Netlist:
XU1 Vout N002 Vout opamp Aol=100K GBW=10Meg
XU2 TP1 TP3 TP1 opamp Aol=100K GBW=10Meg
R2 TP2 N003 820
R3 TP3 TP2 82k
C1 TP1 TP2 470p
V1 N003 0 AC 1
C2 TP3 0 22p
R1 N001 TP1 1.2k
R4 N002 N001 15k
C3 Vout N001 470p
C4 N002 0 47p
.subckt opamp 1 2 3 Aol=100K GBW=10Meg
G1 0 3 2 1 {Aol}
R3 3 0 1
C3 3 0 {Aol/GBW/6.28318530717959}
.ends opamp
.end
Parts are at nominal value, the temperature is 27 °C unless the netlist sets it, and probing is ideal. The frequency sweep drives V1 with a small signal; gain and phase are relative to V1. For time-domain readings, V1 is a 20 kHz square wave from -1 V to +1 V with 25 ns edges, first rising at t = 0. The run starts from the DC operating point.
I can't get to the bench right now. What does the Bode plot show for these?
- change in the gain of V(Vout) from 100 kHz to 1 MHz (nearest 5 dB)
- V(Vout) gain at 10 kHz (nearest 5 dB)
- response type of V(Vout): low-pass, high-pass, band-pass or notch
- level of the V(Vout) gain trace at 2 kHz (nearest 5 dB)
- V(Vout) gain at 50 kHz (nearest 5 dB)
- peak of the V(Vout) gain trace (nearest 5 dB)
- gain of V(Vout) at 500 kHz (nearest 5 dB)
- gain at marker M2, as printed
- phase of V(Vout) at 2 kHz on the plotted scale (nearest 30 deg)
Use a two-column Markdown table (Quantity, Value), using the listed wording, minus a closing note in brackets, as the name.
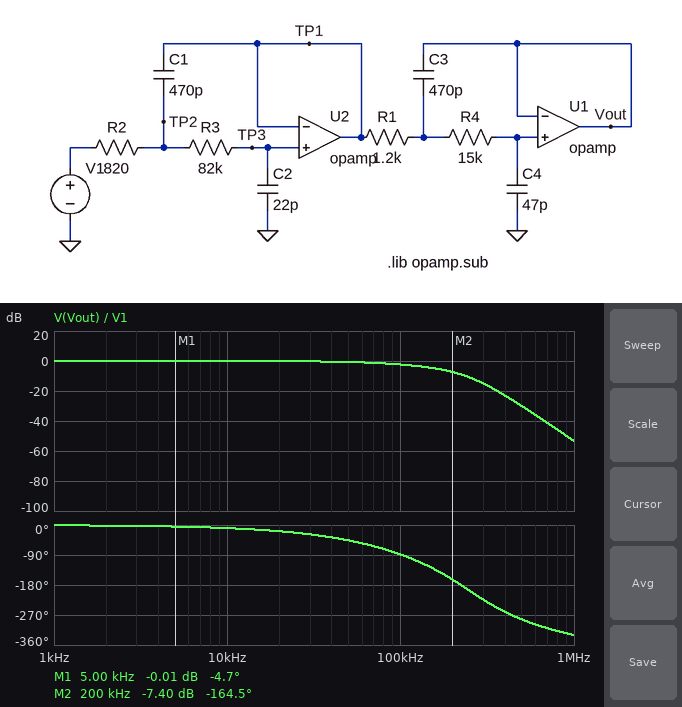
| Quantity | Value |
|---|---|
| change in the gain of V(Vout) from 100 kHz to 1 MHz | -50 dB |
| V(Vout) gain at 10 kHz | 0 dB |
| response type of V(Vout): low-pass, high-pass, band-pass or notch | low-pass |
| level of the V(Vout) gain trace at 2 kHz | 0 dB |
| V(Vout) gain at 50 kHz | 0 dB |
| peak of the V(Vout) gain trace | 0 dB |
| gain of V(Vout) at 500 kHz | -30 dB |
| gain at marker M2, as printed | -7.40 dB |
| phase of V(Vout) at 2 kHz on the plotted scale | 0 deg |
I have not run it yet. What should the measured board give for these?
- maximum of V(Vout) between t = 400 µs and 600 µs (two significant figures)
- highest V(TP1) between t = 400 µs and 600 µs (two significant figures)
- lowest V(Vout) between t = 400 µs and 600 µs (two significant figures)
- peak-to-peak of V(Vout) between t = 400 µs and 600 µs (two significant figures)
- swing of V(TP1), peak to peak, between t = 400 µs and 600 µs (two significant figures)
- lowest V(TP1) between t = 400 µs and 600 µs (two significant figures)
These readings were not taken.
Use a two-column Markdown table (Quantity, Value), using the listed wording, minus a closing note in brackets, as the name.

| Quantity | Value |
|---|---|
| maximum of V(Vout) between t = 400 µs and 600 µs | 1.0 V |
| highest V(TP1) between t = 400 µs and 600 µs | 1.0 V |
| lowest V(Vout) between t = 400 µs and 600 µs | -1.0 V |
| peak-to-peak of V(Vout) between t = 400 µs and 600 µs | 2.0 V |
| swing of V(TP1), peak to peak, between t = 400 µs and 600 µs | 2.0 V |
| lowest V(TP1) between t = 400 µs and 600 µs | -1.0 V |
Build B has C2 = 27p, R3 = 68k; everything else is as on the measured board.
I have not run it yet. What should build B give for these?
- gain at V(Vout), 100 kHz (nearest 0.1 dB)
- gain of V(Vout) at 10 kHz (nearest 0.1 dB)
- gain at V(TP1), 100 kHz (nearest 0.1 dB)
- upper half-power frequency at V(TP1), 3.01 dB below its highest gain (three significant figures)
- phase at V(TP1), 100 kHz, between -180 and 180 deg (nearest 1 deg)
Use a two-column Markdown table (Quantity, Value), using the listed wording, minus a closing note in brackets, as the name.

| Quantity | Value |
|---|---|
| gain at V(Vout), 100 kHz | -2.4 dB |
| gain of V(Vout) at 10 kHz | 0 dB |
| gain at V(TP1), 100 kHz | -2.7 dB |
| upper half-power frequency at V(TP1), 3.01 dB below its highest gain | 106 kHz |
| phase at V(TP1), 100 kHz, between -180 and 180 deg | -59 deg |
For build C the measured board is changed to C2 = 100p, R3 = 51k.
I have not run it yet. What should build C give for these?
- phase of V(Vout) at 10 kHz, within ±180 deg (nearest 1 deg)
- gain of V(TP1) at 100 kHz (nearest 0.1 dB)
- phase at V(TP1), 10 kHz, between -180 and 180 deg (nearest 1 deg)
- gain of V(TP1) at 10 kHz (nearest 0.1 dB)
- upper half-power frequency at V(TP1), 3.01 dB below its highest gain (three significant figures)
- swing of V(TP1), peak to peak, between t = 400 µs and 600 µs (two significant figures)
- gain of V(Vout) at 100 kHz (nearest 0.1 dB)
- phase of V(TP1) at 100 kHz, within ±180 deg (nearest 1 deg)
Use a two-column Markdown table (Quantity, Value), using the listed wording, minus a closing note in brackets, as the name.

| Quantity | Value |
|---|---|
| phase of V(Vout) at 10 kHz, within ±180 deg | -21 deg |
| gain of V(TP1) at 100 kHz | -10.3 dB |
| phase at V(TP1), 10 kHz, between -180 and 180 deg | -18 deg |
| gain of V(TP1) at 10 kHz | -0.4 dB |
| upper half-power frequency at V(TP1), 3.01 dB below its highest gain | 33.1 kHz |
| swing of V(TP1), peak to peak, between t = 400 µs and 600 µs | 2.0 V |
| gain of V(Vout) at 100 kHz | -10.0 dB |
| phase of V(TP1) at 100 kHz, within ±180 deg | -87 deg |
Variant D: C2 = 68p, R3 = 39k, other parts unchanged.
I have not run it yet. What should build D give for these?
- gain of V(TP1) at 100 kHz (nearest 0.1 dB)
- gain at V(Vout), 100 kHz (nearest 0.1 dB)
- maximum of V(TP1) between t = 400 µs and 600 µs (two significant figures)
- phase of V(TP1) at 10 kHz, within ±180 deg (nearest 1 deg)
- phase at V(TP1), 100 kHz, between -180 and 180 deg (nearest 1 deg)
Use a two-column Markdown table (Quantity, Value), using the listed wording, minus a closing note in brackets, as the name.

| Quantity | Value |
|---|---|
| gain of V(TP1) at 100 kHz | -5.1 dB |
| gain at V(Vout), 100 kHz | -4.8 dB |
| maximum of V(TP1) between t = 400 µs and 600 µs | 1.0 V |
| phase of V(TP1) at 10 kHz, within ±180 deg | -10 deg |
| phase at V(TP1), 100 kHz, between -180 and 180 deg | -71 deg |
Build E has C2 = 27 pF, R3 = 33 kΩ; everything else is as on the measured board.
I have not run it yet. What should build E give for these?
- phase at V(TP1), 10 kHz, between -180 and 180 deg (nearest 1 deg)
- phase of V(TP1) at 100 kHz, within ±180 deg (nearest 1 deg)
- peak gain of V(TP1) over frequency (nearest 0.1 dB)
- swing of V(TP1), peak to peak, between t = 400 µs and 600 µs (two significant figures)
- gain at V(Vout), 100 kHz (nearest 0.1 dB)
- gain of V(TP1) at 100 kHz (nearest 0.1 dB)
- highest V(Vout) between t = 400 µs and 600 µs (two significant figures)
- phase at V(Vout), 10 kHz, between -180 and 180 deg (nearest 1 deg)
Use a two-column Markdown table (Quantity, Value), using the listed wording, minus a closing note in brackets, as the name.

| Quantity | Value |
|---|---|
| phase at V(TP1), 10 kHz, between -180 and 180 deg | -3 deg |
| phase of V(TP1) at 100 kHz, within ±180 deg | -34 deg |
| peak gain of V(TP1) over frequency | 0 dB |
| swing of V(TP1), peak to peak, between t = 400 µs and 600 µs | 2.1 V |
| gain at V(Vout), 100 kHz | 0 dB |
| gain of V(TP1) at 100 kHz | -0.3 dB |
| highest V(Vout) between t = 400 µs and 600 µs | 1.2 V |
| phase at V(Vout), 10 kHz, between -180 and 180 deg | -6 deg |
